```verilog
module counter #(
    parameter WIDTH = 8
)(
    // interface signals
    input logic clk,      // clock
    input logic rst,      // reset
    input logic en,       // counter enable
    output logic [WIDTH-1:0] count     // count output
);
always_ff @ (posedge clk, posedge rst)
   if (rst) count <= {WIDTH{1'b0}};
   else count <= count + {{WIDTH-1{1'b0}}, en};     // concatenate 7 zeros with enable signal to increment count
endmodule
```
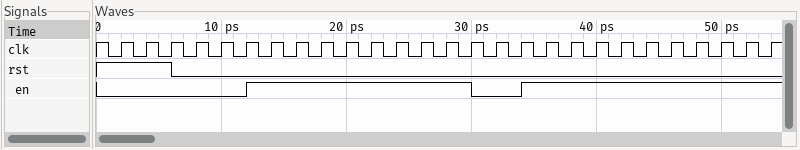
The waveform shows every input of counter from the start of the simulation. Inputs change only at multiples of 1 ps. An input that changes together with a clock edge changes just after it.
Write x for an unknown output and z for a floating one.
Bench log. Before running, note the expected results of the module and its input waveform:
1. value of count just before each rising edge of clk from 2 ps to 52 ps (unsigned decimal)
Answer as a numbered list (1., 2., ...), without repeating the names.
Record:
1. 0, 0, 0, 0, 0, 0, 0, 1, 2, 3, 4, 5, 6, 7, 8, 9, 9, 9, 10, 11, 12, 13, 14, 15, 16, 17
